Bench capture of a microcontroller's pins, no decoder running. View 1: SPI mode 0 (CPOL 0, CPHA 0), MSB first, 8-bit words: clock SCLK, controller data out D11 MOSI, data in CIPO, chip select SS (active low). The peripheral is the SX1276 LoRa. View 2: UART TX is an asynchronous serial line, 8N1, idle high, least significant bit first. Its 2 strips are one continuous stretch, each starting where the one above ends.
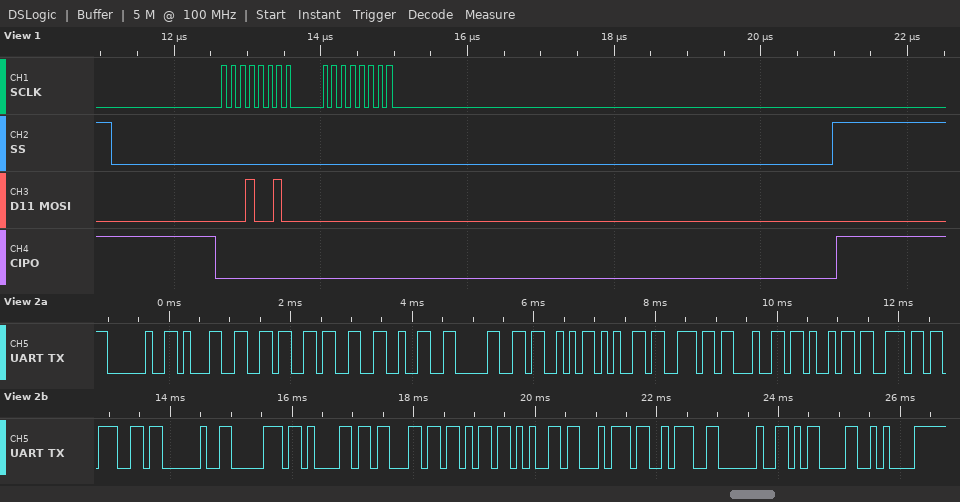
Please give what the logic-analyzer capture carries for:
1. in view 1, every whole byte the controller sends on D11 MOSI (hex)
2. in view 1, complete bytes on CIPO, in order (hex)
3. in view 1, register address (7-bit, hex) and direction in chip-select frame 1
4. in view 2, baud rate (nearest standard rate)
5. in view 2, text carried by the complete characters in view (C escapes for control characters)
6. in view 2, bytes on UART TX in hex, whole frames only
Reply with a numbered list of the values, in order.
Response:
1. 12 00
2. 00 00
3. 0x12 read
4. 9600 baud
5. " 16320Sending packet: \r\n"
6. 20 31 36 33 32 30 53 65 6E 64 69 6E 67 20 70 61 63 6B 65 74 3A 20 0D 0A
